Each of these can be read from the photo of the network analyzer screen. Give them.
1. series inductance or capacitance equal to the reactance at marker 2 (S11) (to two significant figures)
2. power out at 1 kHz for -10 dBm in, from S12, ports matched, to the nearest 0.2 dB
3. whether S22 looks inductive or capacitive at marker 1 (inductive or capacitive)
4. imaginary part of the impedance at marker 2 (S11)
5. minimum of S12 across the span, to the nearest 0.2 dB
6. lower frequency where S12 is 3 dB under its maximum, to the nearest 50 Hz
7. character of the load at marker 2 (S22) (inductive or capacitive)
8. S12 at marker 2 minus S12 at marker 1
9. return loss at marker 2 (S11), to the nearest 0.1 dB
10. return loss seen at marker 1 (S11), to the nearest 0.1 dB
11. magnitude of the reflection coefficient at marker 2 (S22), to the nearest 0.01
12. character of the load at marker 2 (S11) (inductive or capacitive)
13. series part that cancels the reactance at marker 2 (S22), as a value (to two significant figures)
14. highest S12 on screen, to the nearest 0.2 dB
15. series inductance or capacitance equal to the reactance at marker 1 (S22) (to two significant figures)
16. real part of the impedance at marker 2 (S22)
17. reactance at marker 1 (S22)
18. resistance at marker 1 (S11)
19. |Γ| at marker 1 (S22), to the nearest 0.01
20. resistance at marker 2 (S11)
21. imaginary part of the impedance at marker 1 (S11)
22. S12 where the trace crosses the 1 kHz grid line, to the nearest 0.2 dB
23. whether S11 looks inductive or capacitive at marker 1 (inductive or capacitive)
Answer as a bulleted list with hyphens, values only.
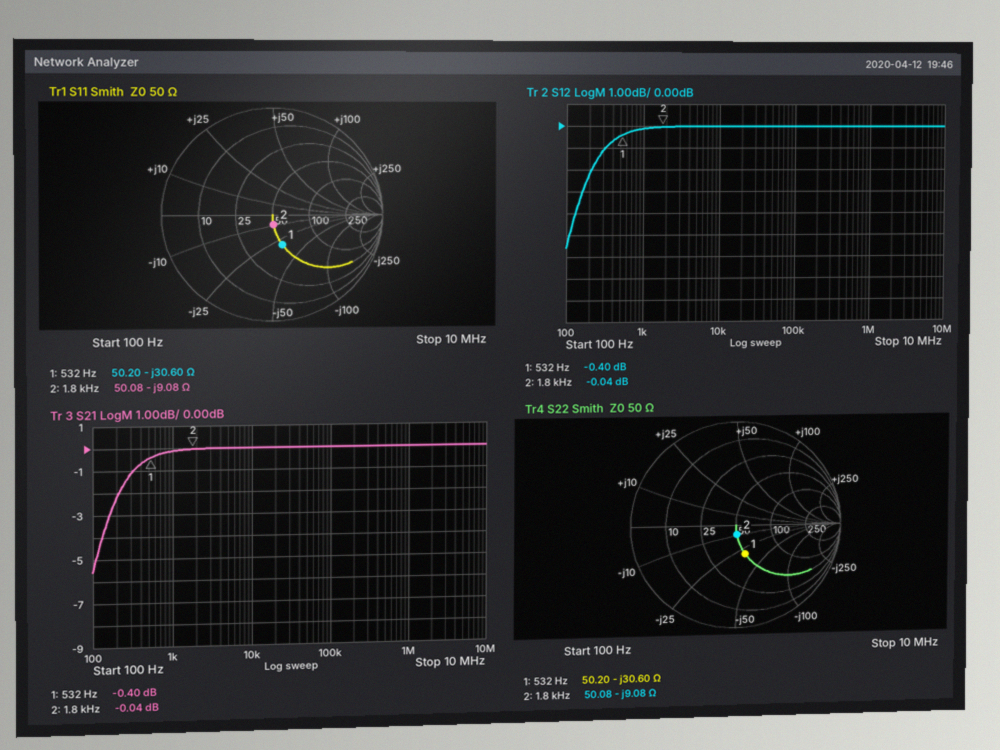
- 9.7 µF
- -10.2 dBm
- capacitive
- -9.08 Ω
- -5.6 dB
- 150 Hz
- capacitive
- 0.36 dB
- 20.9 dB
- 10.7 dB
- 0.09
- capacitive
- 800 µH
- 0.0 dB
- 9.8 µF
- 50.08 Ω
- -30.60 Ω
- 50.20 Ω
- 0.29
- 50.08 Ω
- -30.60 Ω
- -0.2 dB
- capacitive
